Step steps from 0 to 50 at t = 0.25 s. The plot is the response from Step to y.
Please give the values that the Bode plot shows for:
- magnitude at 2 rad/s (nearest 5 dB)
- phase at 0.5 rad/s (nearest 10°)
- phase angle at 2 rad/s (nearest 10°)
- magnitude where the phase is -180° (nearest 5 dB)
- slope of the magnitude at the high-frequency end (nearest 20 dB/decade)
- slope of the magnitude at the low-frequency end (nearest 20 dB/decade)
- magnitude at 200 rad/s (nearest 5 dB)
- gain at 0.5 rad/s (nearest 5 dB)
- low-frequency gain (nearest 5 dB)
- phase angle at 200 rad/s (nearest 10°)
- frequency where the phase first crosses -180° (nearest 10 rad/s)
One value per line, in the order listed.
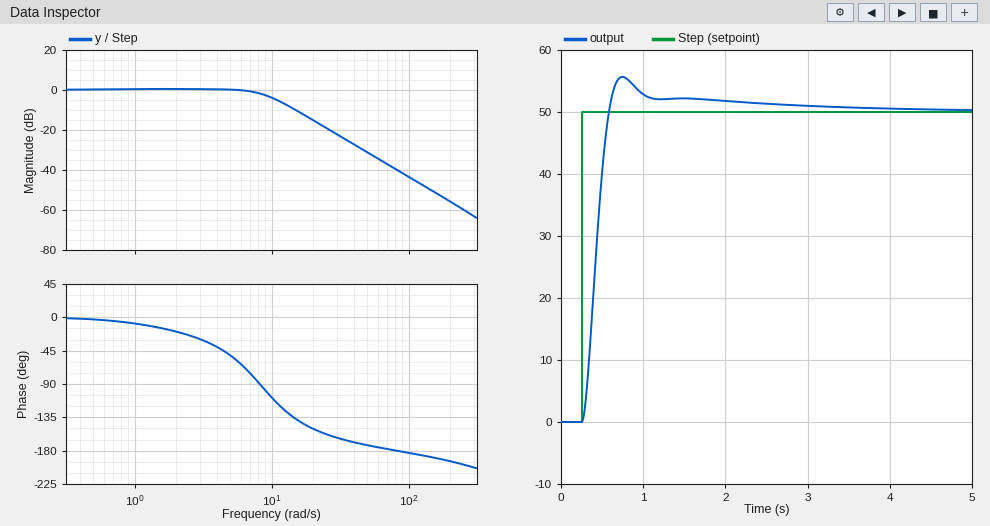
0 dB
0°
-20°
-40 dB
-40 dB/decade
0 dB/decade
-55 dB
0 dB
0 dB
-190°
80 rad/s
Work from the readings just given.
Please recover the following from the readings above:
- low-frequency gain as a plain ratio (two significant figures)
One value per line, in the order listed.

1.0
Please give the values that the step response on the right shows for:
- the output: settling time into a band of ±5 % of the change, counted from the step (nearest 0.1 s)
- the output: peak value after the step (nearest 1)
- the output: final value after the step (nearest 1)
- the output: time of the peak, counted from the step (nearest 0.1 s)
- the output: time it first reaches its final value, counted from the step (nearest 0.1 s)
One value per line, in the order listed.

0.8 s
56
50
0.5 s
0.3 s
